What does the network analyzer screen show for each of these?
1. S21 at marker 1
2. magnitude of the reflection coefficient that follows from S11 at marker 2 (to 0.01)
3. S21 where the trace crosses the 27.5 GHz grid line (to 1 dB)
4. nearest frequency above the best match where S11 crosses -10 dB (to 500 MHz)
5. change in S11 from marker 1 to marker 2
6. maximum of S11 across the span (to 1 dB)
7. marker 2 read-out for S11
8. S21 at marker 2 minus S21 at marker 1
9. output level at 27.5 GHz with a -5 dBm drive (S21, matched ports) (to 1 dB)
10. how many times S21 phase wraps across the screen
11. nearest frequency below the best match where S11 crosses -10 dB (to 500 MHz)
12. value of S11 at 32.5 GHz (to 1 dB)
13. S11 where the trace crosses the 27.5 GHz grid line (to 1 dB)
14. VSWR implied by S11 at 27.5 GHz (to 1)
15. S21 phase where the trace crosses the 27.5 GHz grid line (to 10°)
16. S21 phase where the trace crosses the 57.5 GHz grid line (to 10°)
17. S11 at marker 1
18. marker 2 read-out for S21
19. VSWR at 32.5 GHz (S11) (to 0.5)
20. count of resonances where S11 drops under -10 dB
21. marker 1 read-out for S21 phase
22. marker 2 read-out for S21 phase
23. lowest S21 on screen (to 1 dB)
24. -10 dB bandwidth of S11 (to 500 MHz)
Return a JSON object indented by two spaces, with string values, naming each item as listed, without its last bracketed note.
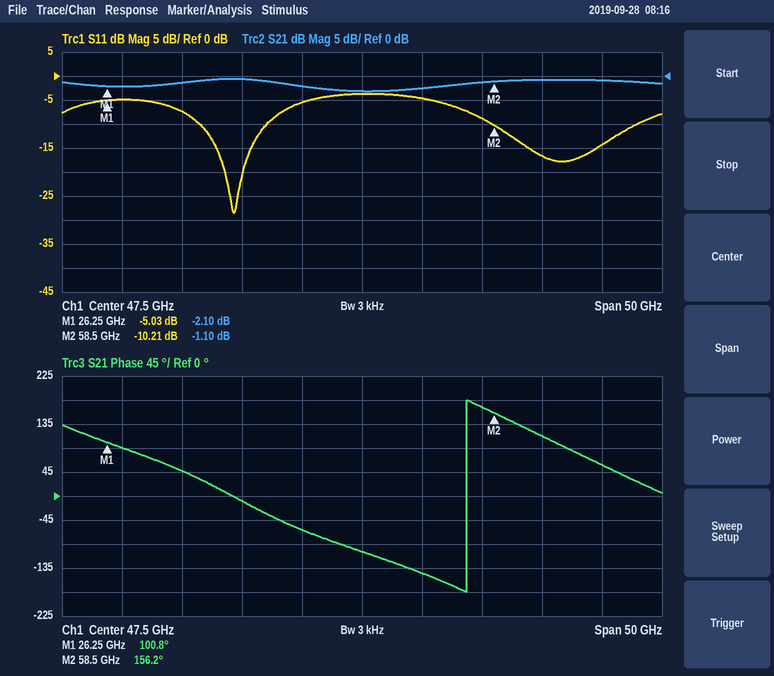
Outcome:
{
  "S21 at marker 1": "-2.10 dB",
  "magnitude of the reflection coefficient that follows from S11 at marker 2": "0.31",
  "S21 where the trace crosses the 27.5 GHz grid line": "-2 dB",
  "nearest frequency above the best match where S11 crosses -10 dB": "39.5 GHz",
  "change in S11 from marker 1 to marker 2": "-5.18 dB",
  "maximum of S11 across the span": "-4 dB",
  "marker 2 read-out for S11": "-10.21 dB",
  "S21 at marker 2 minus S21 at marker 1": "1.00 dB",
  "output level at 27.5 GHz with a -5 dBm drive (S21, matched ports)": "-7 dBm",
  "how many times S21 phase wraps across the screen": "1",
  "nearest frequency below the best match where S11 crosses -10 dB": "34.0 GHz",
  "value of S11 at 32.5 GHz": "-7 dB",
  "S11 where the trace crosses the 27.5 GHz grid line": "-5 dB",
  "VSWR implied by S11 at 27.5 GHz": "4",
  "S21 phase where the trace crosses the 27.5 GHz grid line": "90°",
  "S21 phase where the trace crosses the 57.5 GHz grid line": "170°",
  "S11 at marker 1": "-5.03 dB",
  "marker 2 read-out for S21": "-1.10 dB",
  "VSWR at 32.5 GHz (S11)": "2.5",
  "count of resonances where S11 drops under -10 dB": "2",
  "marker 1 read-out for S21 phase": "100.8°",
  "marker 2 read-out for S21 phase": "156.2°",
  "lowest S21 on screen": "-3 dB",
  "-10 dB bandwidth of S11": "5.5 GHz"
}
